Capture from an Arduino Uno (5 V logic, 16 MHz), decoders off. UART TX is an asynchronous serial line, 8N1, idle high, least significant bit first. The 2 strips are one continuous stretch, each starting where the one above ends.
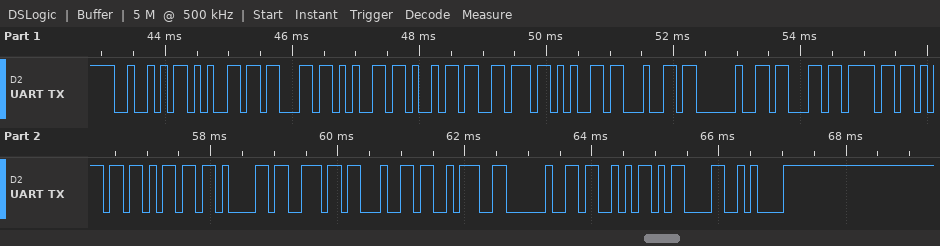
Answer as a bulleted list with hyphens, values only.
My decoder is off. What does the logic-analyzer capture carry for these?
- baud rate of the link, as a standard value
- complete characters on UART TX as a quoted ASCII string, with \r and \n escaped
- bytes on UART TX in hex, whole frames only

- 9600 baud
- "Received command: S\r\n"
- 52 65 63 65 69 76 65 64 20 63 6F 6D 6D 61 6E 64 3A 20 53 0D 0A
